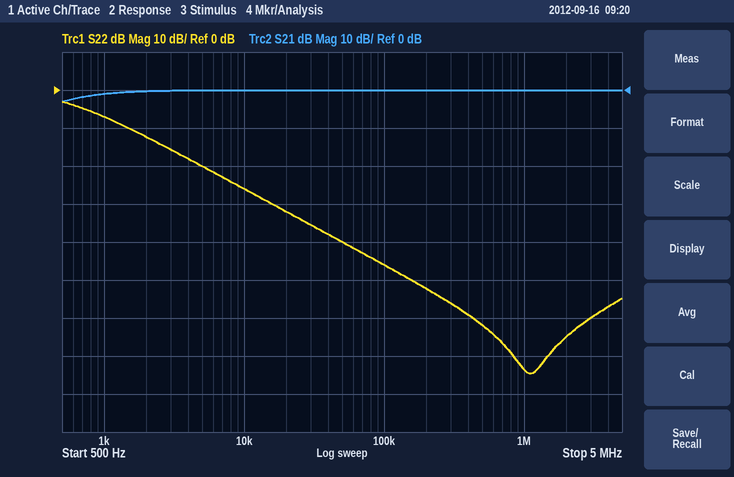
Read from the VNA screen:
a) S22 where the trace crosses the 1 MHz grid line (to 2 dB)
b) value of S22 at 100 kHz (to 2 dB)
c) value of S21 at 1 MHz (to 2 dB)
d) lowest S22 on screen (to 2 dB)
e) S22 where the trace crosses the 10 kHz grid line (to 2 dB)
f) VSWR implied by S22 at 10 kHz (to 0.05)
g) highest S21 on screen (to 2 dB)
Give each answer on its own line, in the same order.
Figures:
-74 dB
-46 dB
0 dB
-74 dB
-26 dB
1.10
0 dB
